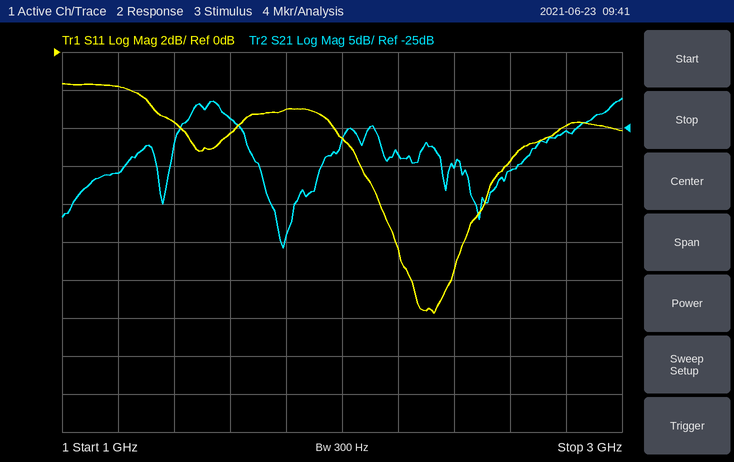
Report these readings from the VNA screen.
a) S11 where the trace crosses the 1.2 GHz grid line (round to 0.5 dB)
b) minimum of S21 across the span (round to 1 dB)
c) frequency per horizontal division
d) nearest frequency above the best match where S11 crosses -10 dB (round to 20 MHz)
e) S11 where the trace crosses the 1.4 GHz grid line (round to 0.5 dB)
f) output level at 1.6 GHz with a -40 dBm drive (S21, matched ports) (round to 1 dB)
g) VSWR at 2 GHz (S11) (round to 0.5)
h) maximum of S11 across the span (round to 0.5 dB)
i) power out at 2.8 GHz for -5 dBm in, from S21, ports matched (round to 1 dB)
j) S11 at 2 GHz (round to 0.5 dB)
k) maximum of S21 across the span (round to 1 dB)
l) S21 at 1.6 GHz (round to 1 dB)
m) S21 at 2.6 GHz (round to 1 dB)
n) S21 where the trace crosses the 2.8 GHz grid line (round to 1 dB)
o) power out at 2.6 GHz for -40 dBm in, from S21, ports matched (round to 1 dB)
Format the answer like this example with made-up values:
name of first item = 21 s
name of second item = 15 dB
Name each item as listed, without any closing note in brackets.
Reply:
S11 where the trace crosses the 1.2 GHz grid line = -2.0 dB
minimum of S21 across the span = -41 dB
frequency per horizontal division = 200 MHz
nearest frequency above the best match where S11 crosses -10 dB = 2.44 GHz
S11 where the trace crosses the 1.4 GHz grid line = -3.5 dB
output level at 1.6 GHz with a -40 dBm drive (S21, matched ports) = -64 dBm
VSWR at 2 GHz (S11) = 4.0
maximum of S11 across the span = -1.5 dB
power out at 2.8 GHz for -5 dBm in, from S21, ports matched = -30 dBm
S11 at 2 GHz = -4.5 dB
maximum of S21 across the span = -21 dB
S21 at 1.6 GHz = -24 dB
S21 at 2.6 GHz = -31 dB
S21 where the trace crosses the 2.8 GHz grid line = -25 dB
power out at 2.6 GHz for -40 dBm in, from S21, ports matched = -71 dBm
